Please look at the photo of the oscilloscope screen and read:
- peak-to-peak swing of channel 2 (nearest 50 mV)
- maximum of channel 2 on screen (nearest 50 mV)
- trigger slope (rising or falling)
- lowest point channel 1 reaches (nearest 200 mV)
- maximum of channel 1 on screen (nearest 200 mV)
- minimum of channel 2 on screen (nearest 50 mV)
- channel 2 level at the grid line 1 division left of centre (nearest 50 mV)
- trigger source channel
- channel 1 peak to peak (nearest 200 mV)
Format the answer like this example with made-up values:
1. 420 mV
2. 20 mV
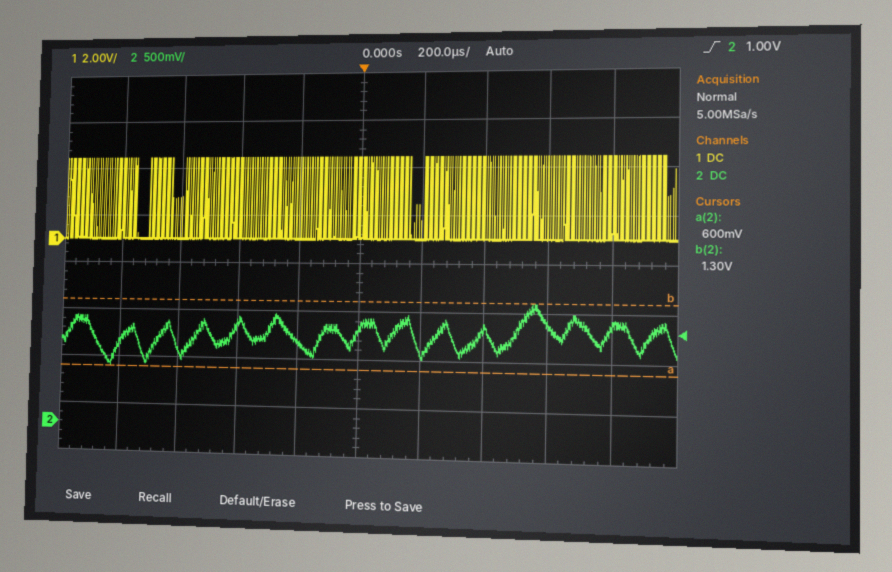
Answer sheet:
1. 700 mV
2. 1.30 V
3. rising
4. 0.0 V
5. 3.4 V
6. 600 mV
7. 900 mV
8. channel 2
9. 3.4 V
